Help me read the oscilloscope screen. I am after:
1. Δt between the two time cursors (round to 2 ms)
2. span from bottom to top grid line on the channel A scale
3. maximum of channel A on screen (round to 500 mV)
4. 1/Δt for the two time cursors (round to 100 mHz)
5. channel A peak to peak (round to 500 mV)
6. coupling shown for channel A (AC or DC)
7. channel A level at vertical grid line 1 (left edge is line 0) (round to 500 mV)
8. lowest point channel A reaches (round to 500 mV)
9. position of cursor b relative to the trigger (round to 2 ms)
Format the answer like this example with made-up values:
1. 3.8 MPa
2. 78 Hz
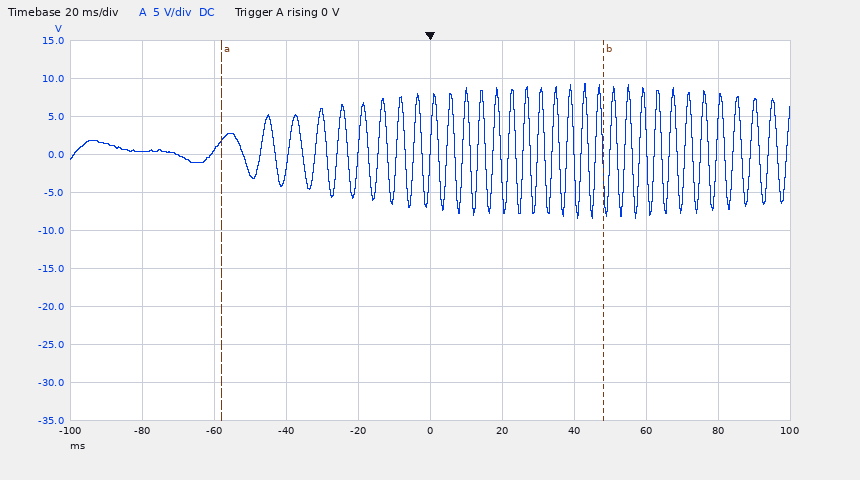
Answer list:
1. 106 ms
2. 50 V
3. 9.5 V
4. 9.4 Hz
5. 18.0 V
6. DC
7. 500 mV
8. -8.5 V
9. +48 ms
